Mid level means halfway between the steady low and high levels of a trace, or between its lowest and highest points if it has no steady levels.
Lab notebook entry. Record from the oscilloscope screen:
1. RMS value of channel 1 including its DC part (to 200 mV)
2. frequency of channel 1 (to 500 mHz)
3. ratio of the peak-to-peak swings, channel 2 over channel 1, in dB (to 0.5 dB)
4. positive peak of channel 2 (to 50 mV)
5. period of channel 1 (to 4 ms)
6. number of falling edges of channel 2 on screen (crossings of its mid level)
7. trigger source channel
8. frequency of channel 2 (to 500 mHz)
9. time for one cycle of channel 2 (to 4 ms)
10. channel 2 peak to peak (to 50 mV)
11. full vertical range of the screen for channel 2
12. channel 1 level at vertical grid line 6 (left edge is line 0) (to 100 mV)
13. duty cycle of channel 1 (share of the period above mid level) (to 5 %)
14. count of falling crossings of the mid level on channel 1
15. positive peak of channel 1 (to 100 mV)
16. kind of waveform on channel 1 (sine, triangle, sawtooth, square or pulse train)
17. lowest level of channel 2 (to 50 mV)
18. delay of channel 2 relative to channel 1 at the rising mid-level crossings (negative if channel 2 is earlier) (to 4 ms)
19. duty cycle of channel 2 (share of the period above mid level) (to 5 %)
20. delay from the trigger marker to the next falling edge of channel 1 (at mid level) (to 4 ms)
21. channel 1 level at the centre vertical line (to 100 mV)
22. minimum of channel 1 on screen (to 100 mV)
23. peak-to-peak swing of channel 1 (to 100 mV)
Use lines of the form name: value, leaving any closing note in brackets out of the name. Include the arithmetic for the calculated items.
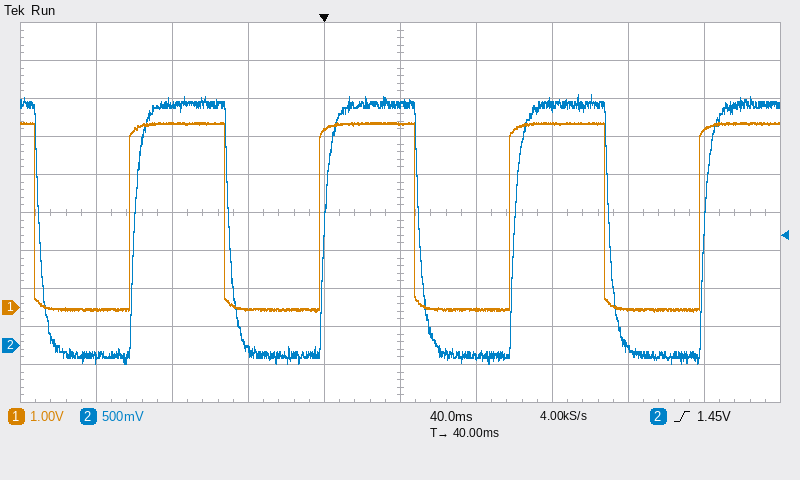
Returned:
RMS value of channel 1 including its DC part: √(0.5 × (4.9 V)² + 0.5 × (-100 mV)²) ≈ 3.47 V, so 3.4 V to the nearest 200 mV
frequency of channel 1: 1 / 100 ms ≈ 10.0 Hz
ratio of the peak-to-peak swings, channel 2 over channel 1, in dB: 20 log10(3.55 V / 5.0 V) ≈ -3.0 dB
positive peak of channel 2: 3.30 V
period of channel 1: 100 ms
number of falling edges of channel 2 on screen: 4
trigger source channel: channel 2
frequency of channel 2: 1 / 100 ms ≈ 10.0 Hz
time for one cycle of channel 2: 100 ms
channel 2 peak to peak: 3.30 V − (-250 mV) = 3.55 V
full vertical range of the screen for channel 2: 5 V
channel 1 level at vertical grid line 6 (left edge is line 0): 0.0 V
duty cycle of channel 1 (share of the period above mid level): 50 %
count of falling crossings of the mid level on channel 1: 4
positive peak of channel 1: 4.9 V
kind of waveform on channel 1: square
lowest level of channel 2: -250 mV
delay of channel 2 relative to channel 1 at the rising mid-level crossings (negative if channel 2 is earlier): +4 ms
duty cycle of channel 2 (share of the period above mid level): 50 %
delay from the trigger marker to the next falling edge of channel 1 (at mid level): 48 ms
channel 1 level at the centre vertical line: 4.8 V
minimum of channel 1 on screen: -100 mV
peak-to-peak swing of channel 1: 4.9 V − (-100 mV) = 5.0 V
